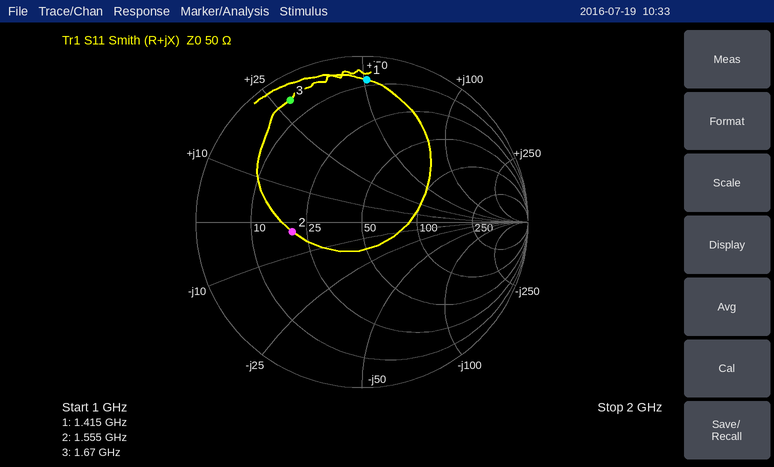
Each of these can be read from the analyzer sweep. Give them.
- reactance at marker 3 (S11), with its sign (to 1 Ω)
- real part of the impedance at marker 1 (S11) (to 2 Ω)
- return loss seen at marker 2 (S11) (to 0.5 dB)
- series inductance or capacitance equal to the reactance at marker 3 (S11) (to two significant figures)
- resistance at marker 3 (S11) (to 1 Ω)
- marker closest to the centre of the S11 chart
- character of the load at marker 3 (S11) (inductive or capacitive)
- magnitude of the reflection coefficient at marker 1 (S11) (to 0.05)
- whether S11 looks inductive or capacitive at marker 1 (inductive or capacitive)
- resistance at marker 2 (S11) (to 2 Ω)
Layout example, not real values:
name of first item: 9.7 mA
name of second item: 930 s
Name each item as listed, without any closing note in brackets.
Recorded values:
reactance at marker 3 (S11), with its sign: +28 Ω
real part of the impedance at marker 1 (S11): 8 Ω
return loss seen at marker 2 (S11): 7.5 dB
series inductance or capacitance equal to the reactance at marker 3 (S11): 2.7 nH
resistance at marker 3 (S11): 5 Ω
marker closest to the centre of the S11 chart: marker 2
character of the load at marker 3 (S11): inductive
magnitude of the reflection coefficient at marker 1 (S11): 0.85
whether S11 looks inductive or capacitive at marker 1: inductive
resistance at marker 2 (S11): 20 Ω
